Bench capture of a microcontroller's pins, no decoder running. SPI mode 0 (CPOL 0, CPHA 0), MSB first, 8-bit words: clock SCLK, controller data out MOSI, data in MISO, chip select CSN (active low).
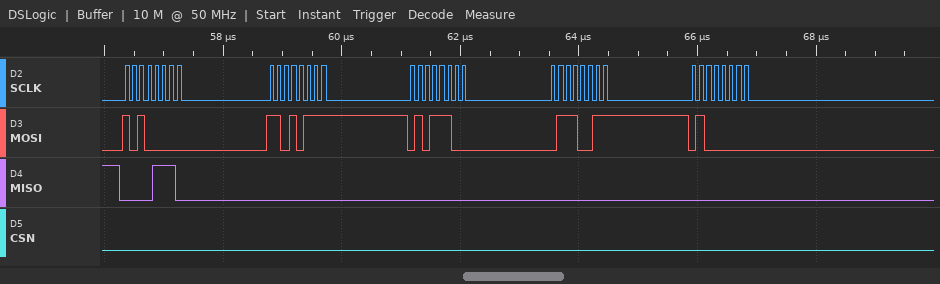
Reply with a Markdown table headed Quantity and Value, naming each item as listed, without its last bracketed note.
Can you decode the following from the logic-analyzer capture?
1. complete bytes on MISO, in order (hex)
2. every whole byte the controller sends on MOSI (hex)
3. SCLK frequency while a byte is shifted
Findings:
| Quantity | Value |
|---|---|
| complete bytes on MISO, in order | 0E 00 00 00 00 |
| every whole byte the controller sends on MOSI | A0 D7 5C 73 40 |
| SCLK frequency while a byte is shifted | 8 MHz |
